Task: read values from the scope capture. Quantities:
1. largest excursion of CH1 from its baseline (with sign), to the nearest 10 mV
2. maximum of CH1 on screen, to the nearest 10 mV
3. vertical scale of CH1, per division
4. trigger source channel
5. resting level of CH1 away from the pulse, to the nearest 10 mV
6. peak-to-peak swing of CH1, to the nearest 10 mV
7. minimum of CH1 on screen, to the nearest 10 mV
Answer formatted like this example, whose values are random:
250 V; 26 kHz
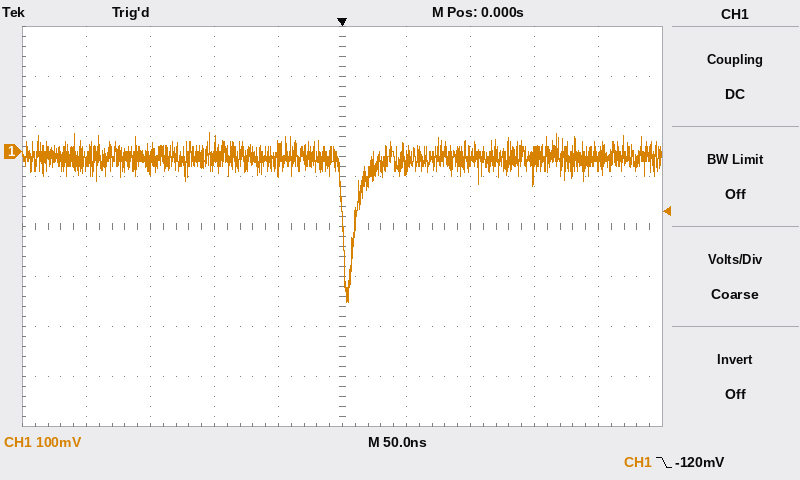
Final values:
-290 mV; 40 mV; 100 mV; CH1; -10 mV; 340 mV; -300 mV
